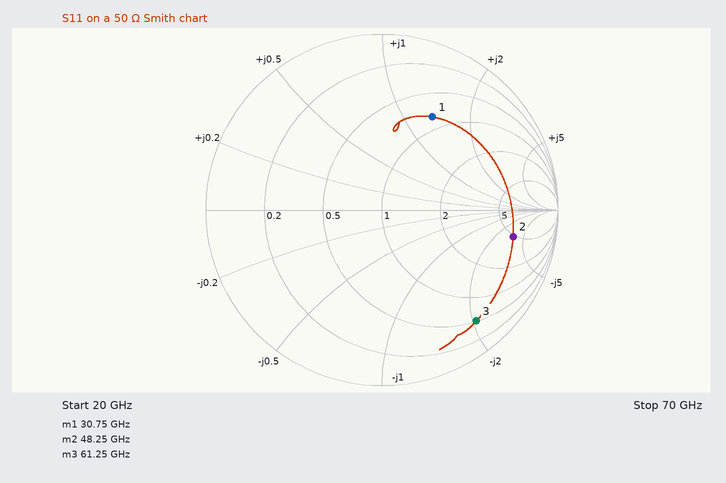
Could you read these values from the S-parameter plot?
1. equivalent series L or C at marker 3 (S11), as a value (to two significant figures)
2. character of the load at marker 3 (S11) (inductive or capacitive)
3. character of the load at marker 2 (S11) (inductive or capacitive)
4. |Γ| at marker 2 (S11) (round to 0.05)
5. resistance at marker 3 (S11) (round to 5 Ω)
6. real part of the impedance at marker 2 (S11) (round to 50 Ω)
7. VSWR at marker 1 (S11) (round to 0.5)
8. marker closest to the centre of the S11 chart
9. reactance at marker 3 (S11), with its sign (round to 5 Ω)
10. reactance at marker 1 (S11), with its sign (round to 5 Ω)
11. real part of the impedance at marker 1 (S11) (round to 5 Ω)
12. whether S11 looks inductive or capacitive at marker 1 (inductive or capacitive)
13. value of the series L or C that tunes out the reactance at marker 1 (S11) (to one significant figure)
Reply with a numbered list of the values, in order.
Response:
1. 25 fF
2. capacitive
3. capacitive
4. 0.75
5. 25 Ω
6. 250 Ω
7. 4.0
8. marker 1
9. -105 Ω
10. +65 Ω
11. 40 Ω
12. inductive
13. 80 fF
